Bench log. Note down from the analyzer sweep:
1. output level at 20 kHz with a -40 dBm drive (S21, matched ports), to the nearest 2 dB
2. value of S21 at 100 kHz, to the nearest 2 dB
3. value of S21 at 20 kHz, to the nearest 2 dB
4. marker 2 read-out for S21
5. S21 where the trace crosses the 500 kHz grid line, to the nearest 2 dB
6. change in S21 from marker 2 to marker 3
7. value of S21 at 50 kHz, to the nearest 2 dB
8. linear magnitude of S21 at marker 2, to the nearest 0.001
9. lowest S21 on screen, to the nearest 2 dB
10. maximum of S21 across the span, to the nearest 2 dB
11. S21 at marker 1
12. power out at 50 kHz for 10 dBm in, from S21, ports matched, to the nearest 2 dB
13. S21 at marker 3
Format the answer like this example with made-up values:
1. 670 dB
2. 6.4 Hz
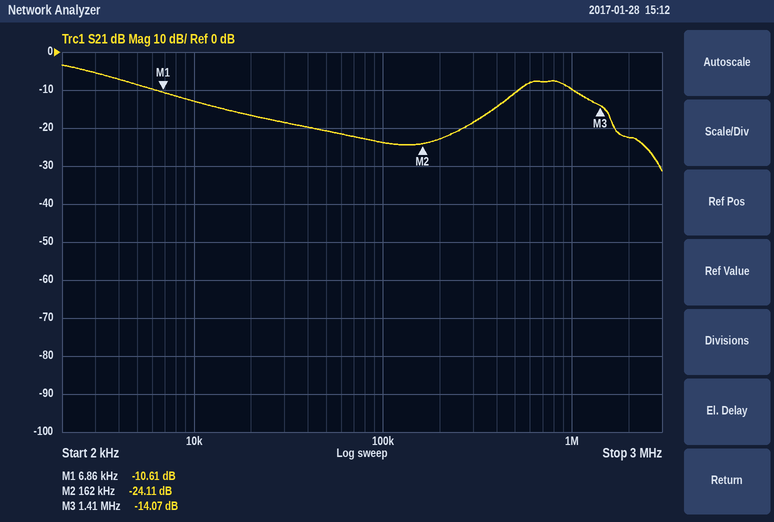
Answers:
1. -56 dBm
2. -24 dB
3. -16 dB
4. -24.11 dB
5. -10 dB
6. 10.04 dB
7. -20 dB
8. 0.062
9. -32 dB
10. -4 dB
11. -10.61 dB
12. -10 dBm
13. -14.07 dB
